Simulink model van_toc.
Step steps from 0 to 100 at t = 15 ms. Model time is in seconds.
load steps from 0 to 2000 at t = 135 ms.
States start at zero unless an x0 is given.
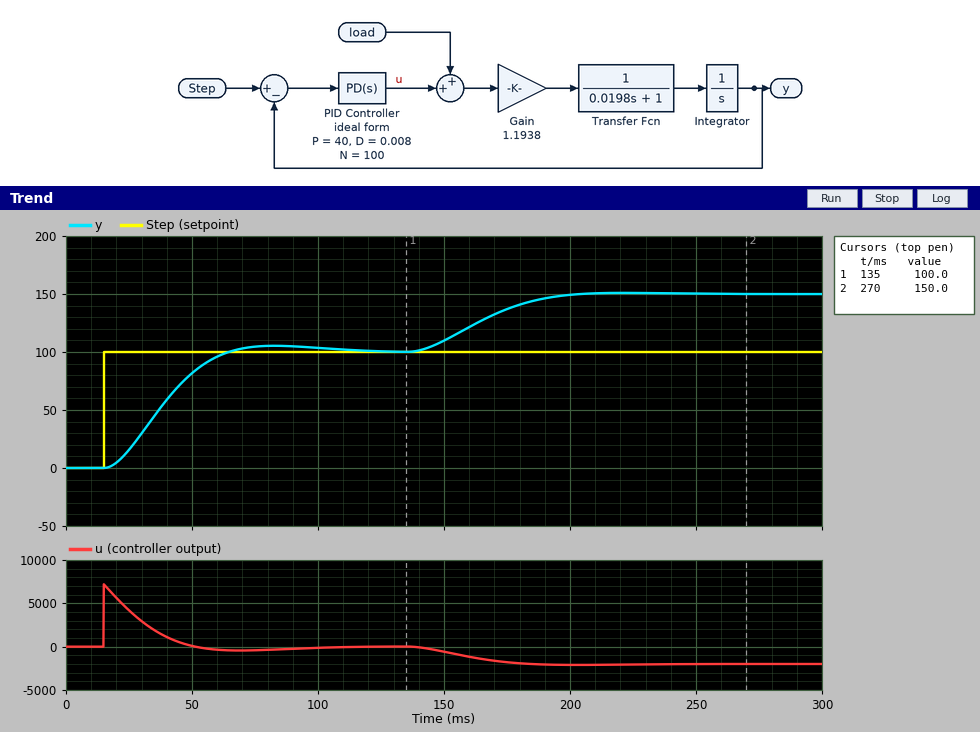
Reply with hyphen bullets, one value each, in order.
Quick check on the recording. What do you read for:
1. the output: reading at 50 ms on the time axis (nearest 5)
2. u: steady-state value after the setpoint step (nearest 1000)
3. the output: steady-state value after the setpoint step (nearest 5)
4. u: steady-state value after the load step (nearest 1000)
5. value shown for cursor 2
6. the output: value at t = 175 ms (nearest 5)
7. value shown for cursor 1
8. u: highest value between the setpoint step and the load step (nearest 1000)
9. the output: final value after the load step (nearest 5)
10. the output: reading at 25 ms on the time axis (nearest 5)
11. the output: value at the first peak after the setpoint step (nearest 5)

- 80
- 0
- 100
- -2000
- 150.0
- 135
- 100.0
- 7000
- 150
- 15
- 105
